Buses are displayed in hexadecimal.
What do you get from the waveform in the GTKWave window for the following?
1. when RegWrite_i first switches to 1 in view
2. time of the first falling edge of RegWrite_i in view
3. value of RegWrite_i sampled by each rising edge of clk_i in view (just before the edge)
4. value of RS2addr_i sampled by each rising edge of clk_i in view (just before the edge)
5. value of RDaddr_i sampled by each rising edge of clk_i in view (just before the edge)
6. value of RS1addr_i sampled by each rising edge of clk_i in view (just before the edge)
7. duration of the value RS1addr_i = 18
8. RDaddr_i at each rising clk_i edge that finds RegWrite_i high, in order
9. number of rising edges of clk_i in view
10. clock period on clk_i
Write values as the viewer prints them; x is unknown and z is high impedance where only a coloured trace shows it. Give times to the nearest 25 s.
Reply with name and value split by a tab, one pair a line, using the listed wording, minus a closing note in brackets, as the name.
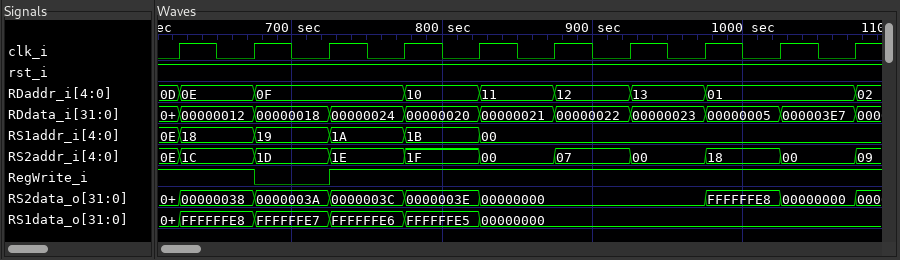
when RegWrite_i first switches to 1 in view	725 s
time of the first falling edge of RegWrite_i in view	675 s
value of RegWrite_i sampled by each rising edge of clk_i in view	1 1 0 1 1 1 1 1 1 1
value of RS2addr_i sampled by each rising edge of clk_i in view	0E, 1C, 1D, 1E, 1F, 00, 07, 00, 18, 00
value of RDaddr_i sampled by each rising edge of clk_i in view	0D, 0E, 0F, 0F, 10, 11, 12, 13, 01, 01
value of RS1addr_i sampled by each rising edge of clk_i in view	0E, 18, 19, 1A, 1B, 00, 00, 00, 00, 00
duration of the value RS1addr_i = 18	50 s
RDaddr_i at each rising clk_i edge that finds RegWrite_i high, in order	0D, 0E, 0F, 10, 11, 12, 13, 01, 01
number of rising edges of clk_i in view	10
clock period on clk_i	50 s
